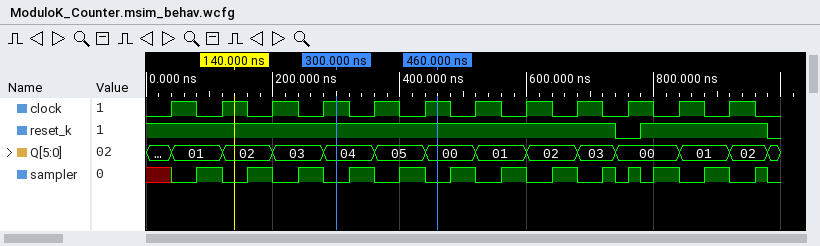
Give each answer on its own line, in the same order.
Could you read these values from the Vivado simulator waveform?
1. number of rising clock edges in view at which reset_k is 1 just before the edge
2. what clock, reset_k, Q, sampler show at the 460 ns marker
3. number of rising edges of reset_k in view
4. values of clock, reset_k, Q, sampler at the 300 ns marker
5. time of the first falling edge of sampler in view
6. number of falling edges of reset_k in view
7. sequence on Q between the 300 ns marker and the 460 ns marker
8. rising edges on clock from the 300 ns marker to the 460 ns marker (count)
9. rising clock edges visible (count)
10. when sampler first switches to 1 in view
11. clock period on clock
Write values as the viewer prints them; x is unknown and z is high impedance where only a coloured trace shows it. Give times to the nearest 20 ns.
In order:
11
clock=1, reset_k=1, Q=00, sampler=0
1
clock=1, reset_k=1, Q=04, sampler=0
120 ns
2
04, 05, 00
2
12
80 ns
80 ns
